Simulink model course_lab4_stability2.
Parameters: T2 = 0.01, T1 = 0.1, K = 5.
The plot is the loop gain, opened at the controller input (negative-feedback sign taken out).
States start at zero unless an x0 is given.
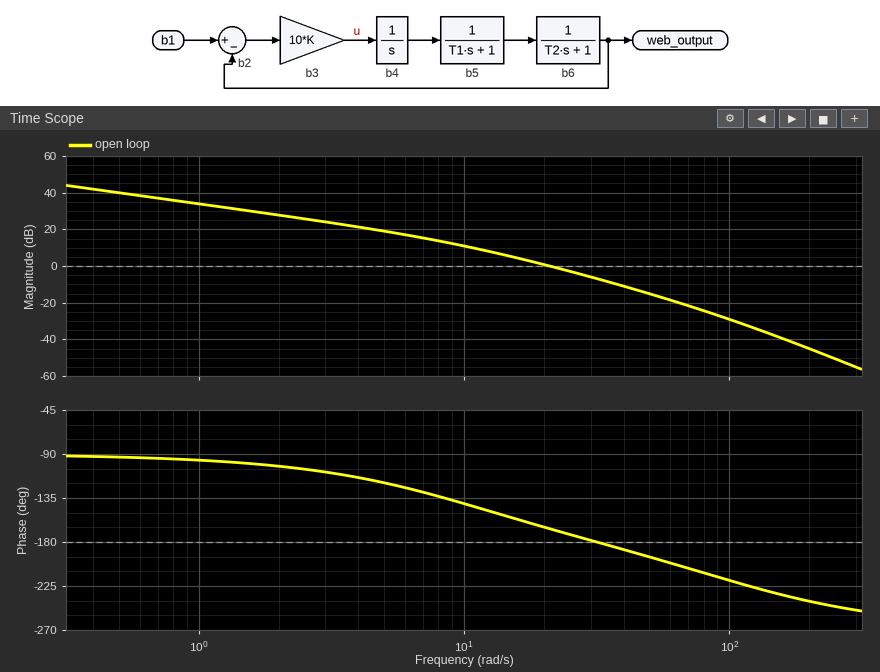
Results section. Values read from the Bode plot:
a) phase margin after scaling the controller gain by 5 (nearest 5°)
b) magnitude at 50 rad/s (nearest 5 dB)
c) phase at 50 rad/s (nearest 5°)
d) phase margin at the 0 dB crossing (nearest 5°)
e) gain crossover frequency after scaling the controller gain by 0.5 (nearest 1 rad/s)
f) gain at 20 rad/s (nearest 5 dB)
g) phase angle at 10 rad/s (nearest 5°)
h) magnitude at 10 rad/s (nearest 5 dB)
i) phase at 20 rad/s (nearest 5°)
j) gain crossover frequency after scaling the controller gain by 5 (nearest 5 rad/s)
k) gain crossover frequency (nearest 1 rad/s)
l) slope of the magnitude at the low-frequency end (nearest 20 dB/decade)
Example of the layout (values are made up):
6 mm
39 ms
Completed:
-15°
-15 dB
-195°
15°
14 rad/s
0 dB
-140°
10 dB
-165°
45 rad/s
21 rad/s
-20 dB/decade
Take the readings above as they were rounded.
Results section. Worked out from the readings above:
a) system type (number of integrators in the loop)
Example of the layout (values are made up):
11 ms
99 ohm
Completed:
1
